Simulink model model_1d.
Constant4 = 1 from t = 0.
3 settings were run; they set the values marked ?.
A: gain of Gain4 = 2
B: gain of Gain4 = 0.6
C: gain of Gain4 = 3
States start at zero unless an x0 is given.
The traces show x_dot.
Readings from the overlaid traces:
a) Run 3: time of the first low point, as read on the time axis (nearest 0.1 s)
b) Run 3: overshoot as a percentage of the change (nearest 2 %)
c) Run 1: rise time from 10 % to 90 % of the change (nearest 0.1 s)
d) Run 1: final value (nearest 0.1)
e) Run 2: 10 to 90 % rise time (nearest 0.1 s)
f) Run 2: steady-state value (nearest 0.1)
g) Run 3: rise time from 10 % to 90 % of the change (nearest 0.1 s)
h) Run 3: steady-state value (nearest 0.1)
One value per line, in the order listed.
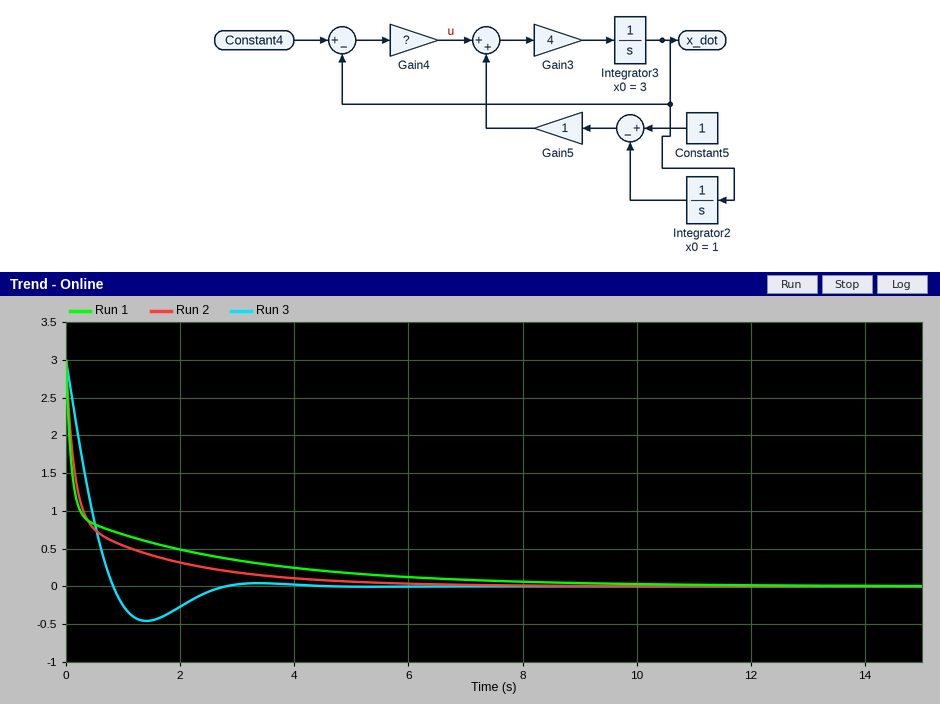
1.4 s
16 %
3.4 s
0.0
2.1 s
0.0
0.6 s
0.0
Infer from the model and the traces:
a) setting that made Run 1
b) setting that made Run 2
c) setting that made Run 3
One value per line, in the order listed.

C
A
B
